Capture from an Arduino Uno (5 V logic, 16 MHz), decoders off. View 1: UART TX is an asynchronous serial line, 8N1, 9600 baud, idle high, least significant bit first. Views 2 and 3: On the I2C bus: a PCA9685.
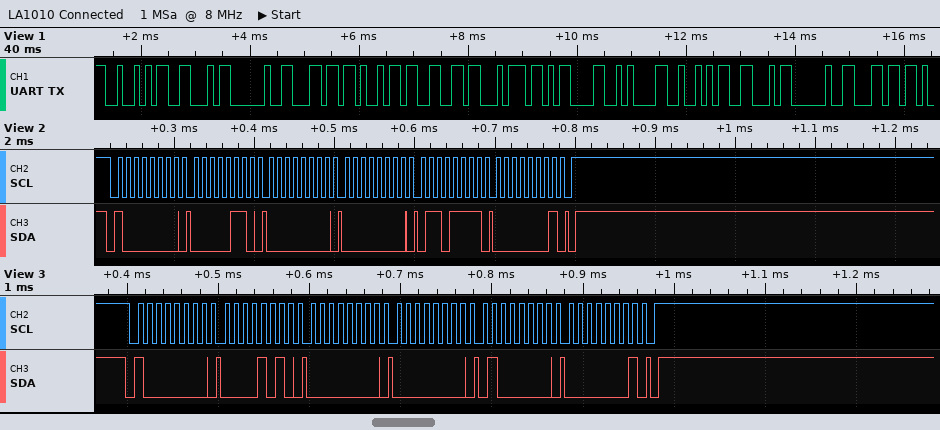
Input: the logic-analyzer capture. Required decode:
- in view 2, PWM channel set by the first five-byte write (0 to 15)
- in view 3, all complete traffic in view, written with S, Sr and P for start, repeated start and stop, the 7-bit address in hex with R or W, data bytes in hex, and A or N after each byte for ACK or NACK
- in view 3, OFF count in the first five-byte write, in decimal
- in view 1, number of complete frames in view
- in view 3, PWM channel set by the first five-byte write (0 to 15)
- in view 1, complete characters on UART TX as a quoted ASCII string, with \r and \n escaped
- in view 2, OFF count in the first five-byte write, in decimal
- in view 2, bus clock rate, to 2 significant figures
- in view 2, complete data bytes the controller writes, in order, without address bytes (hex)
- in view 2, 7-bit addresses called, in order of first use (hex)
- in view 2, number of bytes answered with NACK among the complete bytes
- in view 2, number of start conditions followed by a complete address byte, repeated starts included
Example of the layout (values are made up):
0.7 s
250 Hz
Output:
0
S 40W A 0A A 00 A 00 A 40 A 01 A P
320
13
1
"RF lift\r\nRF l"
367
100 kHz
06 00 00 6F 01
0x40
0
1
